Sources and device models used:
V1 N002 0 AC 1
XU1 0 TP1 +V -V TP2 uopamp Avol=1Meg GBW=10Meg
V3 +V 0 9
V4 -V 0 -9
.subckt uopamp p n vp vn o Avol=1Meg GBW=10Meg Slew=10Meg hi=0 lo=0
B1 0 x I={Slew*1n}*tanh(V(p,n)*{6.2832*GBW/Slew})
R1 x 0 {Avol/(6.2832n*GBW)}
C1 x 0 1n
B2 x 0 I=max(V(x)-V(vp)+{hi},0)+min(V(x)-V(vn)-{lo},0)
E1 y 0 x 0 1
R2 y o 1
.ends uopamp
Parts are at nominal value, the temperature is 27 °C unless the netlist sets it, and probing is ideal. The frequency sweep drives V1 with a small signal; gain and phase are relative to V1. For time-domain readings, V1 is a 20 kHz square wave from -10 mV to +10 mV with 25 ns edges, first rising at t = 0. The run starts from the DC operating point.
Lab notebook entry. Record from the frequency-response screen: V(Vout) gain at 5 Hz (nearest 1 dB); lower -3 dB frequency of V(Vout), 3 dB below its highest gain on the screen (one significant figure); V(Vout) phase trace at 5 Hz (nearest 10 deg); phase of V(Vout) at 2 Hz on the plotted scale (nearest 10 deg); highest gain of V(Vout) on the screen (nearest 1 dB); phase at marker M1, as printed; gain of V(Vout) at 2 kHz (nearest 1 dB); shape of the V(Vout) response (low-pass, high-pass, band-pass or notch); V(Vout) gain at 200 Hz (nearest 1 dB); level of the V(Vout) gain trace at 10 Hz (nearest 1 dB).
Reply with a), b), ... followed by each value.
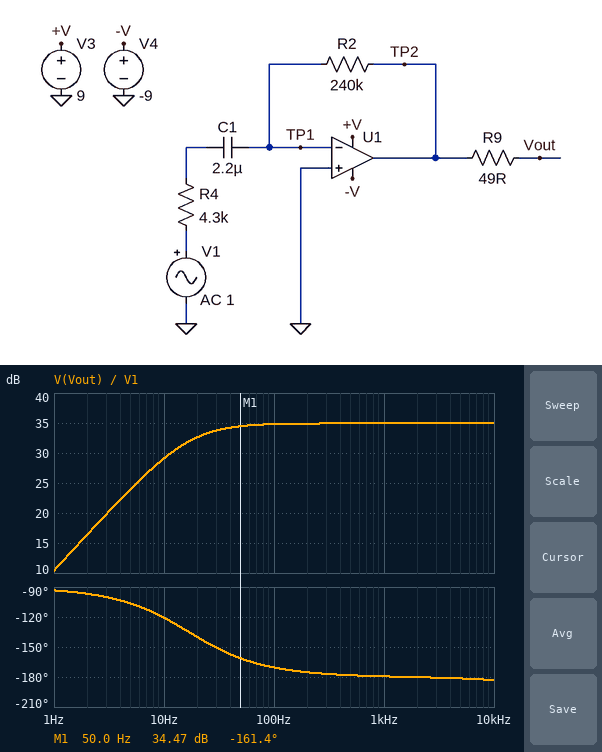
a) 24 dB
b) 20 Hz
c) -110 deg
d) -100 deg
e) 35 dB
f) -161.4 deg
g) 35 dB
h) high-pass
i) 35 dB
j) 29 dB
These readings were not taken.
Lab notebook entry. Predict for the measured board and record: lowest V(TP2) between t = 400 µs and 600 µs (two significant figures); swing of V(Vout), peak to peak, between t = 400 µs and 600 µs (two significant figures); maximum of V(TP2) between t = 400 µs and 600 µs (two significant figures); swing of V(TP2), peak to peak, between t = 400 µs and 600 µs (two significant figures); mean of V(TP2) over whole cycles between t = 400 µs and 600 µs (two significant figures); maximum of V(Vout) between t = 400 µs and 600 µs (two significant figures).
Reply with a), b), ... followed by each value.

a) -1.1 V
b) 1.1 V
c) 34 mV
d) 1.1 V
e) -530 mV
f) 34 mV
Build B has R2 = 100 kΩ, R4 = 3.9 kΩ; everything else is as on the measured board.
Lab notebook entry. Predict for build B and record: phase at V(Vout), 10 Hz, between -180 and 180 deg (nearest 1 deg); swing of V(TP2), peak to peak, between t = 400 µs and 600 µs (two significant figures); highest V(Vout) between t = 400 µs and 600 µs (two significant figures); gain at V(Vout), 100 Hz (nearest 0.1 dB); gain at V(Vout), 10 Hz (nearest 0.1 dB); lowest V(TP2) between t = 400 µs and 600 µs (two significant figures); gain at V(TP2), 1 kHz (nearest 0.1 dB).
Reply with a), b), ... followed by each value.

a) -118 deg
b) 520 mV
c) 17 mV
d) 28.0 dB
e) 21.7 dB
f) -500 mV
g) 28.2 dB
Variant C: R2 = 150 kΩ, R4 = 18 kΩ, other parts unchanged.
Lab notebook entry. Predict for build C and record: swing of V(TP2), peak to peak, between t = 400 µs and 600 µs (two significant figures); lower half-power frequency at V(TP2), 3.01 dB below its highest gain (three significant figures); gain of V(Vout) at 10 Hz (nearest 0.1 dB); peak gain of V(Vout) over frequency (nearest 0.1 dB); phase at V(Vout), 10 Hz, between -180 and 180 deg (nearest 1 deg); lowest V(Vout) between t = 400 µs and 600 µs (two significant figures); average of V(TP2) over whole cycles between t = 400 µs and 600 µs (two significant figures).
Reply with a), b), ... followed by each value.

a) 170 mV
b) 4.02 Hz
c) 17.8 dB
d) 18.4 dB
e) -158 deg
f) -170 mV
g) -82 mV
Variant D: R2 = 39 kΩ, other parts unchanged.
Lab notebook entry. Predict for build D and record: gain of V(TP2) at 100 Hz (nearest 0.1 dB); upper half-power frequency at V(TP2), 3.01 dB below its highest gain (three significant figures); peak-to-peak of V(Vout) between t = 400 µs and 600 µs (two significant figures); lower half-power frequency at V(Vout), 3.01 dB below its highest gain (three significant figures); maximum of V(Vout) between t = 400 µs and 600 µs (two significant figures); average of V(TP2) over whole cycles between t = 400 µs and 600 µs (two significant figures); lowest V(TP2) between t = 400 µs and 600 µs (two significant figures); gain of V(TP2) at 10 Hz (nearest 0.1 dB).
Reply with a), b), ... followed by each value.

a) 19.0 dB
b) 993 kHz
c) 180 mV
d) 16.8 Hz
e) 5.6 mV
f) -86 mV
g) -180 mV
h) 13.3 dB
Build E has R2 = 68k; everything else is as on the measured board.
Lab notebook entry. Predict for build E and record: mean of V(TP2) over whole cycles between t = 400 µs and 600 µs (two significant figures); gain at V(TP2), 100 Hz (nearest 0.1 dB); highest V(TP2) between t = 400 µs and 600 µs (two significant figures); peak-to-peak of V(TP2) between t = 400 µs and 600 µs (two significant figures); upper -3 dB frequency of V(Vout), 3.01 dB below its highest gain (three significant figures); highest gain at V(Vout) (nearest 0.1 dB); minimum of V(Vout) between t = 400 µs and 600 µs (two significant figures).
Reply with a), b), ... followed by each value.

a) -150 mV
b) 23.9 dB
c) 9.7 mV
d) 320 mV
e) 595 kHz
f) 24.0 dB
g) -310 mV
